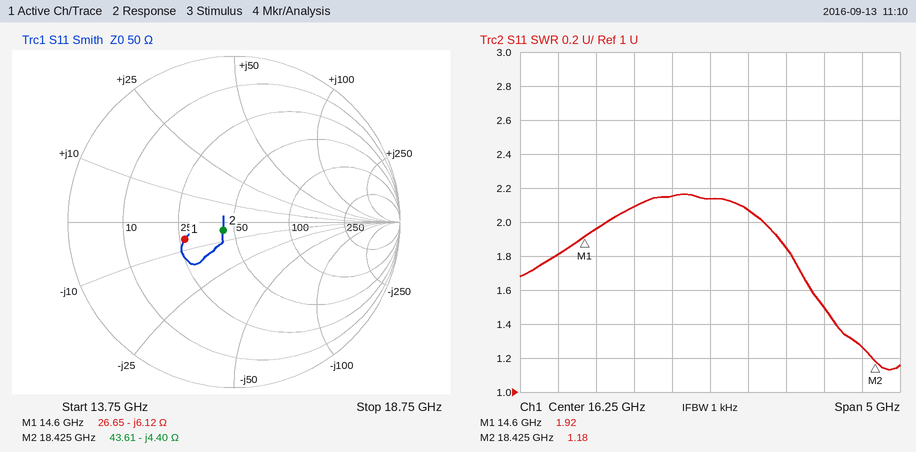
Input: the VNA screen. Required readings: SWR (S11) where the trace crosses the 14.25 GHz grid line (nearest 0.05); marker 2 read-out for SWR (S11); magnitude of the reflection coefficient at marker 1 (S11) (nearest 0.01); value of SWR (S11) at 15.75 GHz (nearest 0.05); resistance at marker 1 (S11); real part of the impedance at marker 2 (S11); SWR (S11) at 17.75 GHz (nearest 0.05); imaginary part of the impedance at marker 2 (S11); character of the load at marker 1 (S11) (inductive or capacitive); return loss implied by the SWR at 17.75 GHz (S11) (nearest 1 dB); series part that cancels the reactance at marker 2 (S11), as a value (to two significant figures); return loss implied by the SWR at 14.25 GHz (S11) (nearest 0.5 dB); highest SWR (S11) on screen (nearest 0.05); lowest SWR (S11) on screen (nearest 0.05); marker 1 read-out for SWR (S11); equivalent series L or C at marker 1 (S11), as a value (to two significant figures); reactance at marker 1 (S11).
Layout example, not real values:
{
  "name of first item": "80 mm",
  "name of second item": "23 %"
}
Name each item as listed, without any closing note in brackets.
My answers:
{
  "SWR (S11) where the trace crosses the 14.25 GHz grid line": "1.80",
  "marker 2 read-out for SWR": "1.18",
  "magnitude of the reflection coefficient at marker 1 (S11)": "0.31",
  "value of SWR (S11) at 15.75 GHz": "2.15",
  "resistance at marker 1": "26.65 Ω",
  "real part of the impedance at marker 2": "43.61 Ω",
  "SWR (S11) at 17.75 GHz": "1.50",
  "imaginary part of the impedance at marker 2": "-4.40 Ω",
  "character of the load at marker 1 (S11)": "capacitive",
  "return loss implied by the SWR at 17.75 GHz (S11)": "14 dB",
  "series part that cancels the reactance at marker 2 (S11), as a value": "38 pH",
  "return loss implied by the SWR at 14.25 GHz (S11)": "11.0 dB",
  "highest SWR (S11) on screen": "2.15",
  "lowest SWR (S11) on screen": "1.15",
  "marker 1 read-out for SWR": "1.92",
  "equivalent series L or C at marker 1 (S11), as a value": "1.8 pF",
  "reactance at marker 1": "-6.12 Ω"
}
